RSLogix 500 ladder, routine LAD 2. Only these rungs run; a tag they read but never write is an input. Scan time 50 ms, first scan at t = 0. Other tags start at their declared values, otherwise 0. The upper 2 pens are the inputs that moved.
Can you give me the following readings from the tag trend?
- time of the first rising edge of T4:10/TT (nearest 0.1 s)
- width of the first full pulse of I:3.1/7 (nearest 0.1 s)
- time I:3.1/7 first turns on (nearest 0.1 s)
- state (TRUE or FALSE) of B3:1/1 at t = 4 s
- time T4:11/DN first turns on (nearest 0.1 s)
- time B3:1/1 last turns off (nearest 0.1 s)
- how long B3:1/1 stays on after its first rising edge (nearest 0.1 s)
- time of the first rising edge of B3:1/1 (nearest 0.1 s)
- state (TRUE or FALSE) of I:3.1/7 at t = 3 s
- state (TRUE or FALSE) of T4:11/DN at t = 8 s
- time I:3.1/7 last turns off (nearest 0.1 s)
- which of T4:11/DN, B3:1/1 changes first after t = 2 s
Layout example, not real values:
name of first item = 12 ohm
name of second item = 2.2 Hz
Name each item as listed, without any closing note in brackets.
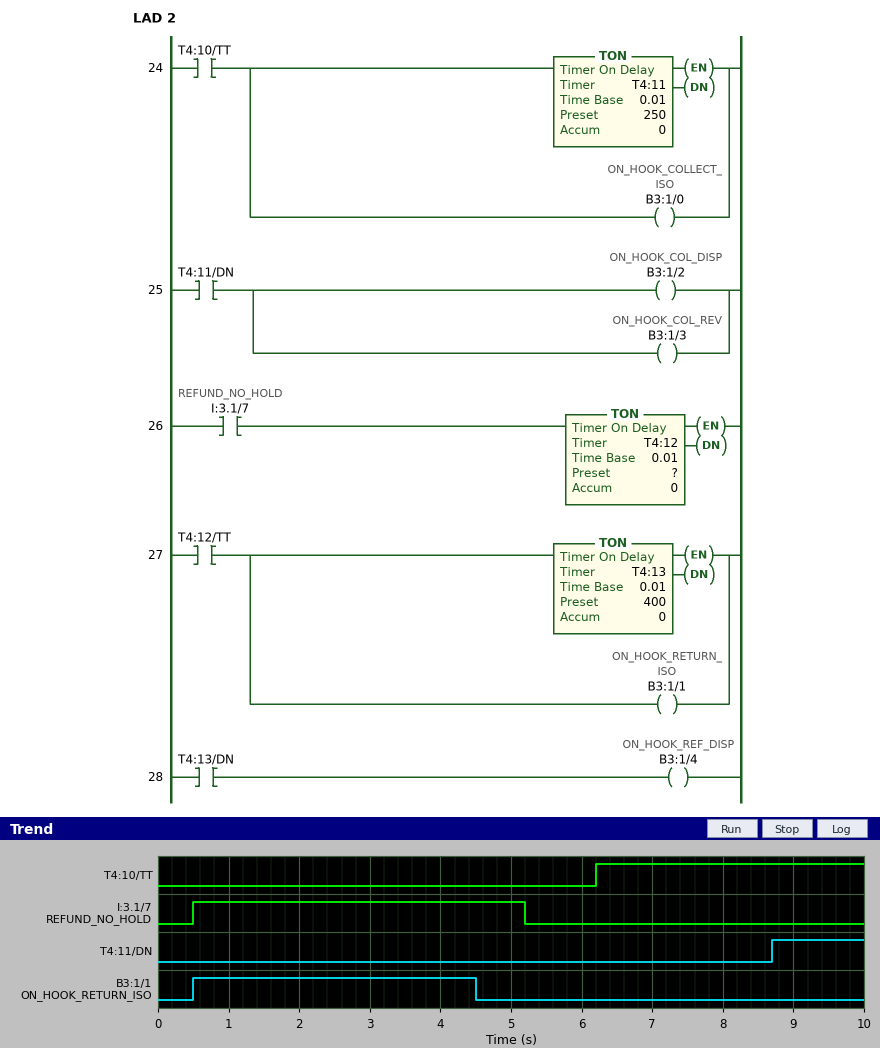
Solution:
time of the first rising edge of T4:10/TT = 6.2 s
width of the first full pulse of I:3.1/7 = 4.7 s
time I:3.1/7 first turns on = 0.5 s
state (TRUE or FALSE) of B3:1/1 at t = 4 s = TRUE
time T4:11/DN first turns on = 8.7 s
time B3:1/1 last turns off = 4.5 s
how long B3:1/1 stays on after its first rising edge = 4.0 s
time of the first rising edge of B3:1/1 = 0.5 s
state (TRUE or FALSE) of I:3.1/7 at t = 3 s = TRUE
state (TRUE or FALSE) of T4:11/DN at t = 8 s = FALSE
time I:3.1/7 last turns off = 5.2 s
which of T4:11/DN, B3:1/1 changes first after t = 2 s = B3:1/1
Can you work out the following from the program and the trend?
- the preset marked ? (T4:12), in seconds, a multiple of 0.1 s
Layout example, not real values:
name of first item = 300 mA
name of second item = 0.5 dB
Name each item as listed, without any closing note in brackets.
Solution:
the preset marked ? (T4:12), in seconds, a multiple of 0.1 s = 4.0 s
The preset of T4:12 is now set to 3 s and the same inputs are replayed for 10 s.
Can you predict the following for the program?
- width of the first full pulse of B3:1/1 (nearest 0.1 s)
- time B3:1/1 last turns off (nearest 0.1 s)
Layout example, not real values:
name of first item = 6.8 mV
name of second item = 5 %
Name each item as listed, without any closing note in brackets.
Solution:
width of the first full pulse of B3:1/1 = 3.0 s
time B3:1/1 last turns off = 3.5 s
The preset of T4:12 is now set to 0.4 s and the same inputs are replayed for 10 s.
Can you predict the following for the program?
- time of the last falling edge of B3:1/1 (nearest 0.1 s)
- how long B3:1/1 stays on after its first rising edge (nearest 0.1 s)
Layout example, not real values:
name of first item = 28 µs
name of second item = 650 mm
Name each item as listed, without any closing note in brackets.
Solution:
time of the last falling edge of B3:1/1 = 0.9 s
how long B3:1/1 stays on after its first rising edge = 0.4 s
